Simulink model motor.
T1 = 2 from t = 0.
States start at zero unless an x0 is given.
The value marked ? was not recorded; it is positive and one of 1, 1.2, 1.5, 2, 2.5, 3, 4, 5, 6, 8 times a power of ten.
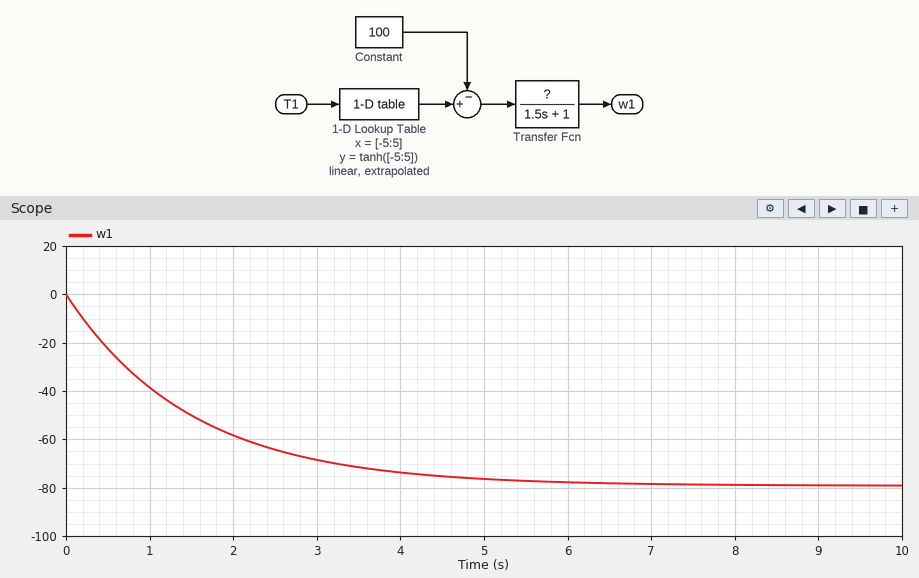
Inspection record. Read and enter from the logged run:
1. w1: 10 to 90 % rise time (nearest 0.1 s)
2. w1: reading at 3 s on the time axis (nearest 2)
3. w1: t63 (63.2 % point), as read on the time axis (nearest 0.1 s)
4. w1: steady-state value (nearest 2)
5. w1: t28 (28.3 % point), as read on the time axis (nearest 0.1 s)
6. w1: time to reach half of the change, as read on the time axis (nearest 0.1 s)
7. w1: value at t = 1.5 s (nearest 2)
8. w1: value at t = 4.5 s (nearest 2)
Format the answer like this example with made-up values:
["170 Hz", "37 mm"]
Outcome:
["3.3 s", "-68", "1.5 s", "-80", "0.5 s", "1.0 s", "-50", "-76"]
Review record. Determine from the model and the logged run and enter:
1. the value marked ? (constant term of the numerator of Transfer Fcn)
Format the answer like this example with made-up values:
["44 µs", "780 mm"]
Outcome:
["0.8"]
